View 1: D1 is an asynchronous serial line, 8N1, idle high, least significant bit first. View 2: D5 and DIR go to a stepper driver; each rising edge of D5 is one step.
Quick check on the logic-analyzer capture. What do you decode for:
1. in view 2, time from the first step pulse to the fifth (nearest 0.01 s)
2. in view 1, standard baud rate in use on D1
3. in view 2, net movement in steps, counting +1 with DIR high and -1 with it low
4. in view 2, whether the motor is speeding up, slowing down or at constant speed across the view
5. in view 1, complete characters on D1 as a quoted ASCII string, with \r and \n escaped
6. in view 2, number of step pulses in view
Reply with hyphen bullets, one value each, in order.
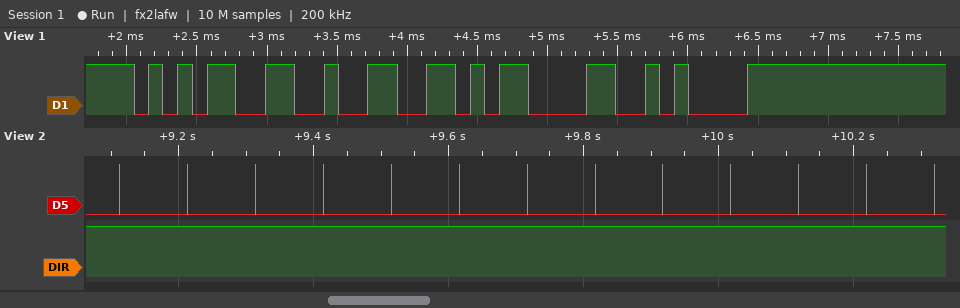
- 0.40 s
- 9600 baud
- +13
- constant speed
- "52\r\n"
- 13
